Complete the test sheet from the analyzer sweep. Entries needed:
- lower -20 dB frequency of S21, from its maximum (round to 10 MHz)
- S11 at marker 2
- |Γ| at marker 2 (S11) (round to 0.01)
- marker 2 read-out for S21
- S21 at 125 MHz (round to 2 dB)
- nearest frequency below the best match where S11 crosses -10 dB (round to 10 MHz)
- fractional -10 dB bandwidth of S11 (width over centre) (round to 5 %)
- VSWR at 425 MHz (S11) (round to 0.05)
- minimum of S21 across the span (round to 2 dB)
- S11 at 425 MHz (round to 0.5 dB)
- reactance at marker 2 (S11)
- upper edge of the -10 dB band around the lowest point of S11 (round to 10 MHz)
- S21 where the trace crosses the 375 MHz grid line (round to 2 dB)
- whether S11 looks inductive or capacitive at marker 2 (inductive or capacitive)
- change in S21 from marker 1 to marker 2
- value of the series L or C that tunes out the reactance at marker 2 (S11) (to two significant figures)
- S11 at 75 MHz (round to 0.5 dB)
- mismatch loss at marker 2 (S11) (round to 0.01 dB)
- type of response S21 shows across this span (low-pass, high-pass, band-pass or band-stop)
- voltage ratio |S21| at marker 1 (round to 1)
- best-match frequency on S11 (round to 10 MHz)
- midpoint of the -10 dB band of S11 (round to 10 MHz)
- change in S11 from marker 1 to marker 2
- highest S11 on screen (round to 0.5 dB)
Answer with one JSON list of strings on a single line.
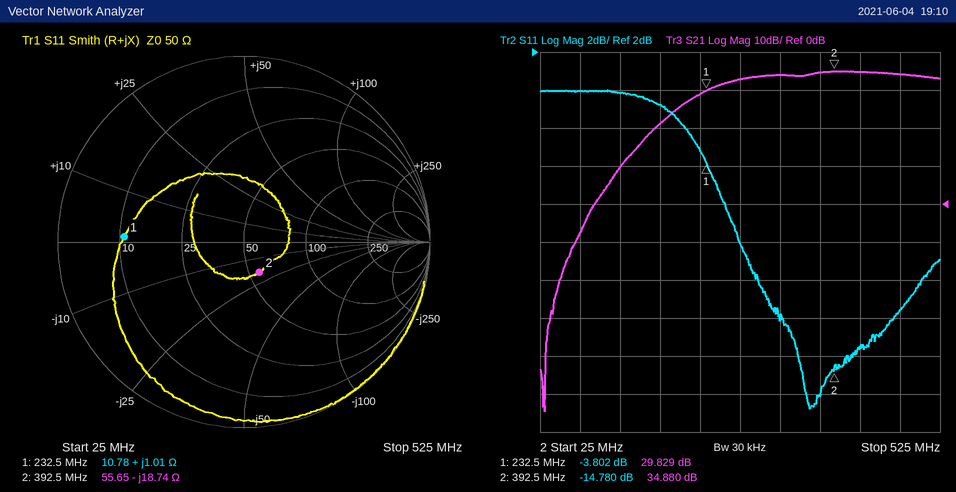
["150 MHz", "-14.780 dB", "0.18", "34.880 dB", "10 dB", "300 MHz", "50 %", "1.55", "-54 dB", "-13.5 dB", "-18.74 Ω", "500 MHz", "34 dB", "capacitive", "5.051 dB", "7.6 nH", "0.0 dB", "0.15 dB", "high-pass", "31", "360 MHz", "400 MHz", "-10.978 dB", "0.0 dB"]
